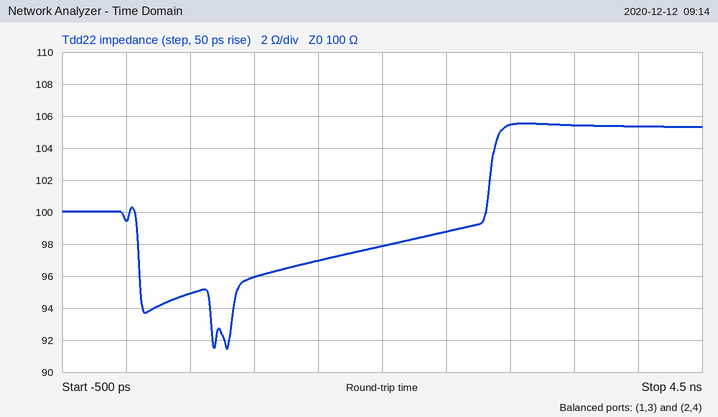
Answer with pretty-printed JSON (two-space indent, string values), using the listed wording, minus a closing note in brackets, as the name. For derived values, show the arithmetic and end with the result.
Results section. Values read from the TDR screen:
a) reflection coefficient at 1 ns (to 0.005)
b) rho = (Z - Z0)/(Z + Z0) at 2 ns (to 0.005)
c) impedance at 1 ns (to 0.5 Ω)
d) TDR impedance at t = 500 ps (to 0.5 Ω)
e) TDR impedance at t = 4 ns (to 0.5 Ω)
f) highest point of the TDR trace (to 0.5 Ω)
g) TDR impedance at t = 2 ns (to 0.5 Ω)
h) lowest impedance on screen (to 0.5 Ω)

{
  "reflection coefficient at 1 ns": "(96 − 100)/(96 + 100) ≈ -0.020",
  "rho = (Z - Z0)/(Z + Z0) at 2 ns": "(98 − 100)/(98 + 100) ≈ -0.010",
  "impedance at 1 ns": "96.0 Ω",
  "TDR impedance at t = 500 ps": "95.0 Ω",
  "TDR impedance at t = 4 ns": "105.5 Ω",
  "highest point of the TDR trace": "105.5 Ω",
  "TDR impedance at t = 2 ns": "98.0 Ω",
  "lowest impedance on screen": "91.5 Ω"
}
